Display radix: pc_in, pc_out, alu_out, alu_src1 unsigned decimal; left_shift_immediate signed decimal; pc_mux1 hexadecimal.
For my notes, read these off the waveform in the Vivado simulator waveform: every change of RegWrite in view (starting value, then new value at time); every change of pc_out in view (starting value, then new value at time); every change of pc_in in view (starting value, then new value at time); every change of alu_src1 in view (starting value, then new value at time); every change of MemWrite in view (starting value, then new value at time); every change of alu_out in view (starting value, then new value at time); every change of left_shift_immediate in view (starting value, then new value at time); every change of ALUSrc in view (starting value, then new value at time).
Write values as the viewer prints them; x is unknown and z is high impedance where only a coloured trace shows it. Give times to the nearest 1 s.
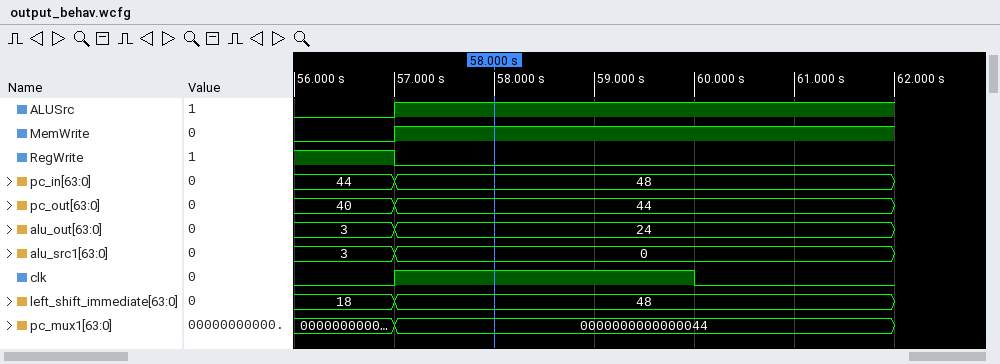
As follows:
1, 0 at 57 s
40, 44 at 57 s
44, 48 at 57 s
3, 0 at 57 s
0, 1 at 57 s
3, 24 at 57 s
18, 48 at 57 s
0, 1 at 57 s
